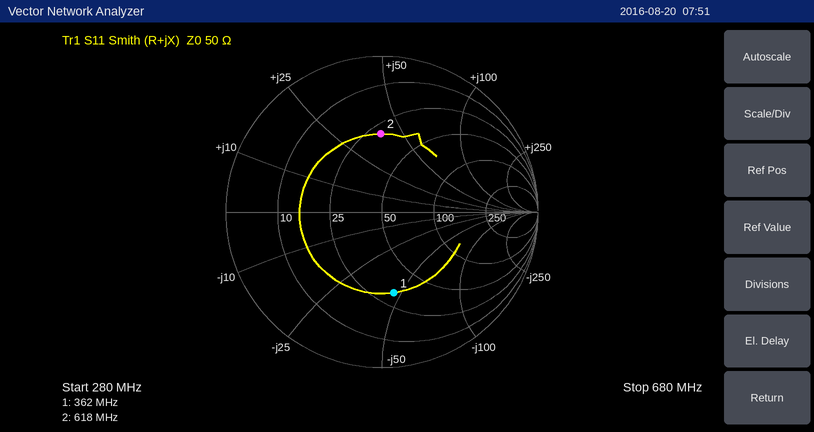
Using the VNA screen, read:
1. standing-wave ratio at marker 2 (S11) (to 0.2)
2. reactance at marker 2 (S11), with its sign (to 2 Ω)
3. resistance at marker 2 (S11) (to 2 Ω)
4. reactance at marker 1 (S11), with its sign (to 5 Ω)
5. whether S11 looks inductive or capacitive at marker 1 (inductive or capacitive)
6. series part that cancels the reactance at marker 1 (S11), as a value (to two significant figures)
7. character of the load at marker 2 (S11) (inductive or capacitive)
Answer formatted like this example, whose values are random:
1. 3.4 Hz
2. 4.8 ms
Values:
1. 3.0
2. +40 Ω
3. 30 Ω
4. -45 Ω
5. capacitive
6. 20 nH
7. inductive
